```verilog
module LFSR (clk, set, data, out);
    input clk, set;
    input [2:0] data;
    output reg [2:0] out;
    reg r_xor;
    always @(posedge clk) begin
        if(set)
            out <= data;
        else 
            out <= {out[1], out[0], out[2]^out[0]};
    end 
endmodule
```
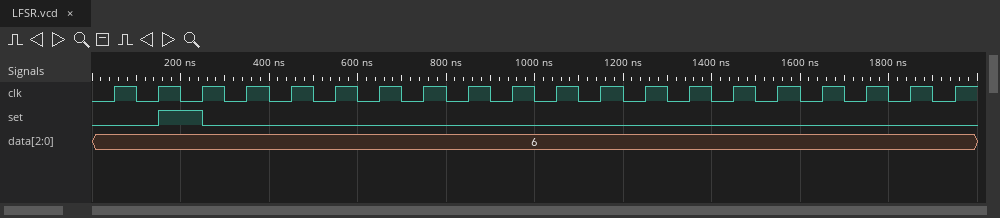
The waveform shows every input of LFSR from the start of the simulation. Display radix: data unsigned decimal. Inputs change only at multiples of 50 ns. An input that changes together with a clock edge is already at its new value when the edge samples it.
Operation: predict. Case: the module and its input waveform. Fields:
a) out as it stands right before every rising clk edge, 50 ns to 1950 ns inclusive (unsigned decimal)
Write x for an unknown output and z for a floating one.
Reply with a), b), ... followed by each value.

a) x, x, 6, 5, 2, 4, 1, 3, 7, 6, 5, 2, 4, 1, 3, 7, 6, 5, 2, 4
